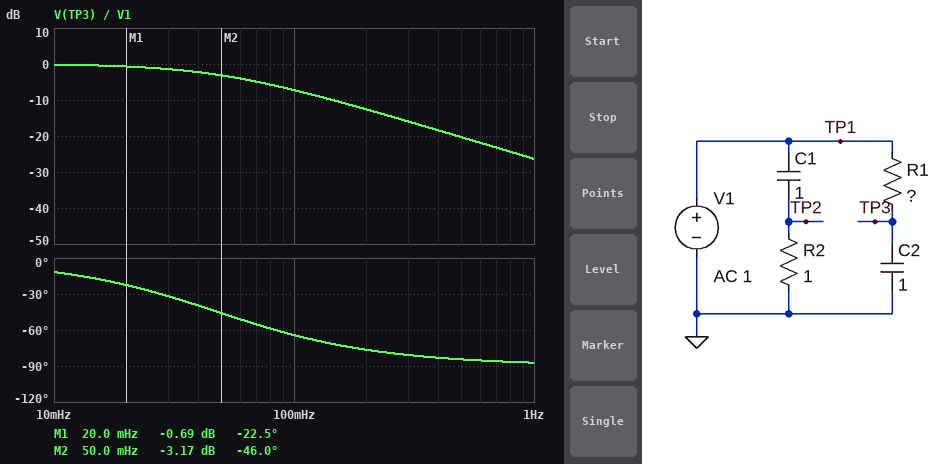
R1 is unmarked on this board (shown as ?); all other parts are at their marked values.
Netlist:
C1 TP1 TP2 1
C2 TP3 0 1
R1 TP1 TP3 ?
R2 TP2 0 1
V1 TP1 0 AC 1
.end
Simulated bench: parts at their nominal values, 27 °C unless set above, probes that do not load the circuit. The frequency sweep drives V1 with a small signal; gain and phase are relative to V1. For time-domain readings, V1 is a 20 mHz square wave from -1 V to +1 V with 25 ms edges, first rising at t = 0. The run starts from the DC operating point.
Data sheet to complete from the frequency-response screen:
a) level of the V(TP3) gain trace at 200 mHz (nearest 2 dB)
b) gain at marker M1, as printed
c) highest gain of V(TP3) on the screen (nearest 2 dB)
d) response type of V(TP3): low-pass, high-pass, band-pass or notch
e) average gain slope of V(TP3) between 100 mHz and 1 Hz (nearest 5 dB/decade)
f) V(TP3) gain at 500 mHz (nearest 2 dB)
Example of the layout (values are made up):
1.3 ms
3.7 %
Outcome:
-12 dB
-0.69 dB
0 dB
low-pass
-20 dB/decade
-20 dB
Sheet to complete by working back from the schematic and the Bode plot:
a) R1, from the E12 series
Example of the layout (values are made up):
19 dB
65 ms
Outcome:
3.3 Ω
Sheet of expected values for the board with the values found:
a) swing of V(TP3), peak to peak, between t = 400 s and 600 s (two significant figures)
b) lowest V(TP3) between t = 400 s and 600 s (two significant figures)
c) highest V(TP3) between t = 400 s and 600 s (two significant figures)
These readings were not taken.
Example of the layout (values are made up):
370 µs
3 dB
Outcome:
2.0 V
-1.0 V
1.0 V
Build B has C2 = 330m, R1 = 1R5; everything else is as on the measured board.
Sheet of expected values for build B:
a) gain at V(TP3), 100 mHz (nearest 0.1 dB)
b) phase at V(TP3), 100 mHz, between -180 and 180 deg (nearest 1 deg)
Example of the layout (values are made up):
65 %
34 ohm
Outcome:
-0.4 dB
-17 deg
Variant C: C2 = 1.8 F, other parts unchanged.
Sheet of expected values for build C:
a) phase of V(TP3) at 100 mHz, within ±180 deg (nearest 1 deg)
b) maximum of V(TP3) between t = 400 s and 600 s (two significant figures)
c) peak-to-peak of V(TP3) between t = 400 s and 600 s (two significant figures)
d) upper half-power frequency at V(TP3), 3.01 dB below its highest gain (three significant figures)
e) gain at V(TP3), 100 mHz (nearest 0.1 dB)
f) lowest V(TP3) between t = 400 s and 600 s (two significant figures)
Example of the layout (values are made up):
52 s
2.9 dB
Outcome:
-75 deg
970 mV
1.9 V
26.8 mHz
-11.7 dB
-970 mV
